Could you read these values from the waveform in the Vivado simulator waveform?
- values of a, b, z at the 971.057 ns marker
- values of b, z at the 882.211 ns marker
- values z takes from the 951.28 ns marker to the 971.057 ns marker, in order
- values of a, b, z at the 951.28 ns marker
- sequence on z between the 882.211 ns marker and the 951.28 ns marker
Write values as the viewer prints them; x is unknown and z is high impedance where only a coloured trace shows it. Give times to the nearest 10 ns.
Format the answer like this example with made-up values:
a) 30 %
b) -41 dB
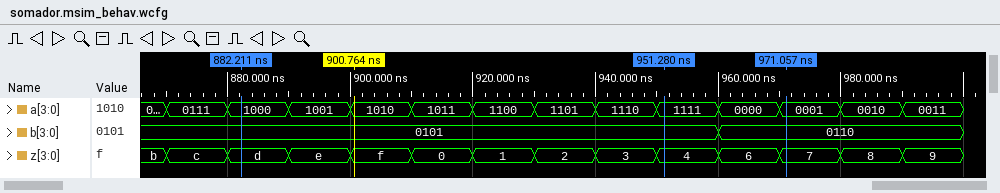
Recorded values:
a) a=0001, b=0110, z=7
b) b=0101, z=d
c) 4, 6, 7
d) a=1111, b=0101, z=4
e) d, e, f, 0, 1, 2, 3, 4
